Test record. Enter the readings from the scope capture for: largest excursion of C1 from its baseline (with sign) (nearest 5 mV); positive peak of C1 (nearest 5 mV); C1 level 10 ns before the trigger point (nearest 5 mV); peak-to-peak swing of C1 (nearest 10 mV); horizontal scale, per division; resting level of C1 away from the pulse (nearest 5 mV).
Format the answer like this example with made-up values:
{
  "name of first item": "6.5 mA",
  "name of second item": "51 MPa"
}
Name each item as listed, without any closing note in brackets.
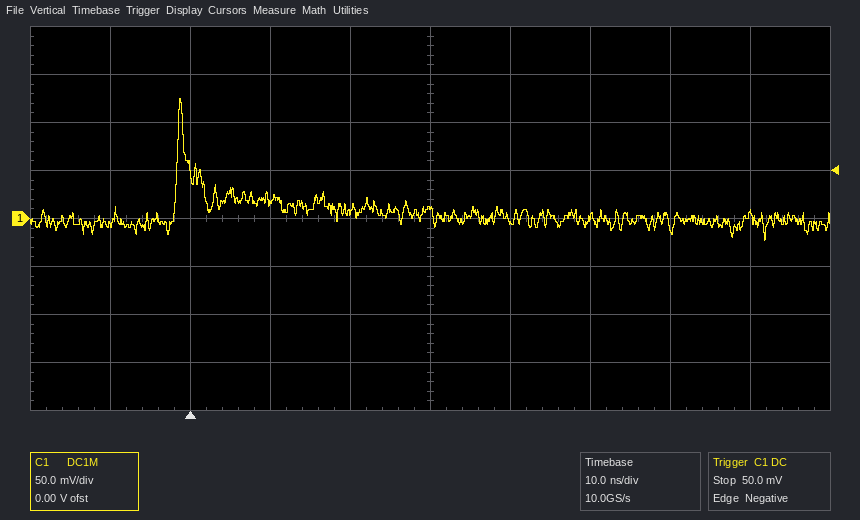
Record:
{
  "largest excursion of C1 from its baseline (with sign)": "+125 mV",
  "positive peak of C1": "125 mV",
  "C1 level 10 ns before the trigger point": "-5 mV",
  "peak-to-peak swing of C1": "150 mV",
  "horizontal scale, per division": "10 ns",
  "resting level of C1 away from the pulse": "0 mV"
}
